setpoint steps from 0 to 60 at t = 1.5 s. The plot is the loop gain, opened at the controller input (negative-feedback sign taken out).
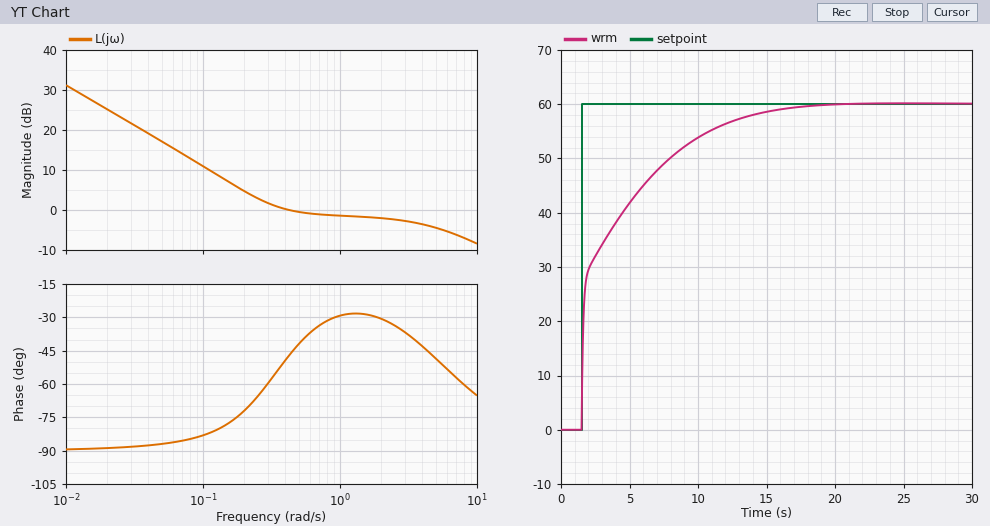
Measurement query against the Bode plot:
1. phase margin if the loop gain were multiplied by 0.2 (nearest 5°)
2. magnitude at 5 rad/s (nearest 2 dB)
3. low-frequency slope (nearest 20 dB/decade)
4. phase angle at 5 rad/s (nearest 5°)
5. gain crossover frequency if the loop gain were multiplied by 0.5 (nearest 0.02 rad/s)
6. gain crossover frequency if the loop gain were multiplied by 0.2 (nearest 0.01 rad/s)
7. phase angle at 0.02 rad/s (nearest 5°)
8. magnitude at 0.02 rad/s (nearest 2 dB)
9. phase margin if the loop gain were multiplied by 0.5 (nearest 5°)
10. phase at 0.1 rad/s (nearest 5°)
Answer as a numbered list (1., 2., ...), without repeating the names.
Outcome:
1. 95°
2. -4 dB
3. -20 dB/decade
4. -50°
5. 0.18 rad/s
6. 0.07 rad/s
7. -90°
8. 26 dB
9. 105°
10. -85°
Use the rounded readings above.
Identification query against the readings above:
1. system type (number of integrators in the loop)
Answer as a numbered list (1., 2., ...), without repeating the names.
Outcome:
1. 1
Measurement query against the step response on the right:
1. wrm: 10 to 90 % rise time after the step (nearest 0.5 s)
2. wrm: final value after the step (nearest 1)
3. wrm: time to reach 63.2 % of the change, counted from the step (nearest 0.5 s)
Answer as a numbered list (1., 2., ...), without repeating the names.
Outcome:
1. 8.5 s
2. 60
3. 2.5 s
